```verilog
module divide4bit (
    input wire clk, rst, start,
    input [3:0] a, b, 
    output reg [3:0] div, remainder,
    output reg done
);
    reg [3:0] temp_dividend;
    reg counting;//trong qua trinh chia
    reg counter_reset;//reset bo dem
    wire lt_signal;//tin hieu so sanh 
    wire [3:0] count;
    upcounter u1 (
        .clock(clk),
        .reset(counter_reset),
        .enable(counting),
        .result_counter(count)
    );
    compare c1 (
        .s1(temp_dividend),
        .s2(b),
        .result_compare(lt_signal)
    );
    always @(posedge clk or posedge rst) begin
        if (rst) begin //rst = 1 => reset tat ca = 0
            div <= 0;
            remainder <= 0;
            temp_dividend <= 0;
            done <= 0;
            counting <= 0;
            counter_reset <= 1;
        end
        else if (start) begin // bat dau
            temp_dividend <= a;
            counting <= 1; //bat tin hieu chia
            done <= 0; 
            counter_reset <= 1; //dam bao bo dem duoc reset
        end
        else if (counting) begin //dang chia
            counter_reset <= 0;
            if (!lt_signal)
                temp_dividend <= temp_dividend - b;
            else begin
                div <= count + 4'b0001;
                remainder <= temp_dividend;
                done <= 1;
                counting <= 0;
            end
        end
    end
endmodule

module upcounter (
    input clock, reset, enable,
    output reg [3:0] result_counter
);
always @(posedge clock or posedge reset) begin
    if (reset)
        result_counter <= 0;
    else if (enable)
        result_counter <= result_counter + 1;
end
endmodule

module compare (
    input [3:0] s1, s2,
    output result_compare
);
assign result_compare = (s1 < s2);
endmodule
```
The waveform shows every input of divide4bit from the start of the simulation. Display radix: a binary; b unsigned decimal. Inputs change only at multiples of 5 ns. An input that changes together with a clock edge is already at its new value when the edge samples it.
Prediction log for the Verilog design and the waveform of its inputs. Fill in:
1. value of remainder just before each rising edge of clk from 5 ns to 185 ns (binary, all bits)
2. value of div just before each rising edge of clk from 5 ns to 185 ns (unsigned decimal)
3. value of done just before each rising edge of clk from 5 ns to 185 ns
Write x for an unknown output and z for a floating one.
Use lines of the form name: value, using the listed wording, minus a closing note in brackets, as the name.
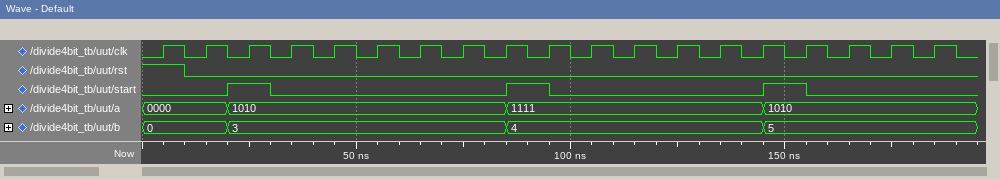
value of remainder just before each rising edge of clk from 5 ns to 185 ns: 0000, 0000, 0000, 0000, 0000, 0000, 0000, 0001, 0001, 0001, 0001, 0001, 0001, 0011, 0011, 0011, 0011, 0011, 0000
value of div just before each rising edge of clk from 5 ns to 185 ns: 0, 0, 0, 0, 0, 0, 0, 3, 3, 3, 3, 3, 3, 3, 3, 3, 3, 3, 2
value of done just before each rising edge of clk from 5 ns to 185 ns: 0 0 0 0 0 0 0 1 1 0 0 0 0 1 1 0 0 0 1
